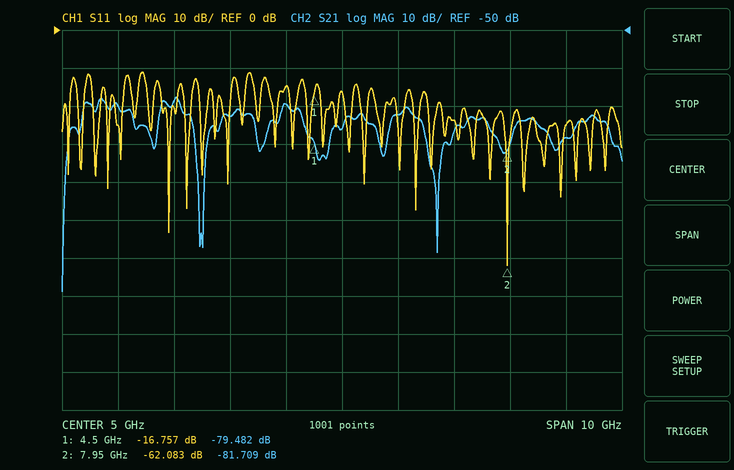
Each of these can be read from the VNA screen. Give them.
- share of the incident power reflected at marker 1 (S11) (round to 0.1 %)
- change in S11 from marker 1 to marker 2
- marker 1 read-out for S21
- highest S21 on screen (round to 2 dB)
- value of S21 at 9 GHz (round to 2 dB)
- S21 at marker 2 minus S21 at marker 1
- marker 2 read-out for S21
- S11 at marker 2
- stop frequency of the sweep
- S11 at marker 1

2.1 %
-45.326 dB
-79.482 dB
-68 dB
-78 dB
-2.227 dB
-81.709 dB
-62.083 dB
10 GHz
-16.757 dB
